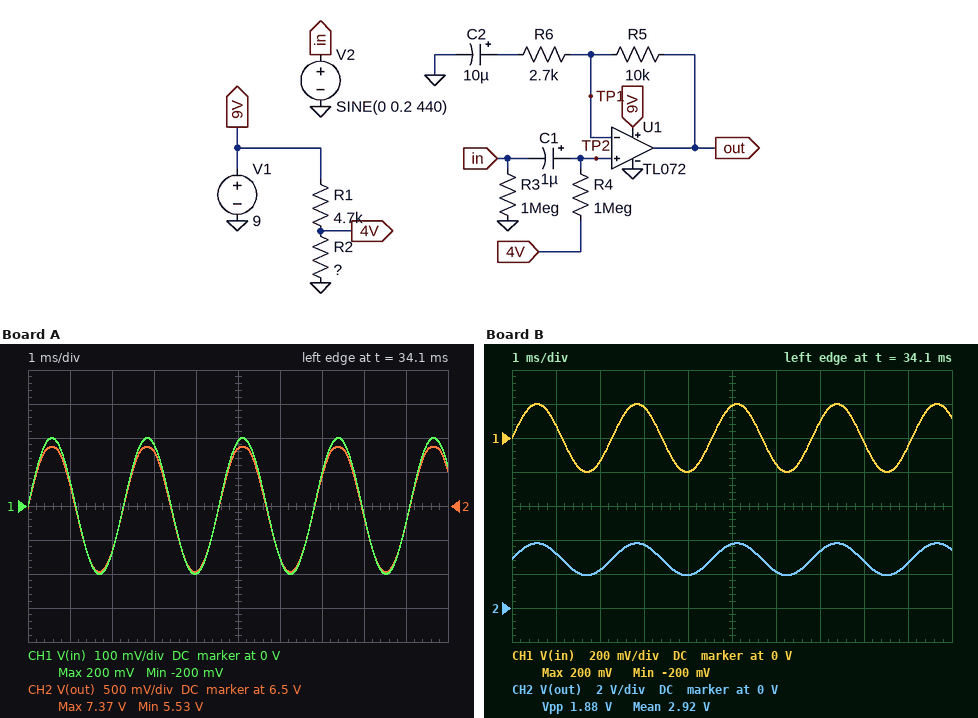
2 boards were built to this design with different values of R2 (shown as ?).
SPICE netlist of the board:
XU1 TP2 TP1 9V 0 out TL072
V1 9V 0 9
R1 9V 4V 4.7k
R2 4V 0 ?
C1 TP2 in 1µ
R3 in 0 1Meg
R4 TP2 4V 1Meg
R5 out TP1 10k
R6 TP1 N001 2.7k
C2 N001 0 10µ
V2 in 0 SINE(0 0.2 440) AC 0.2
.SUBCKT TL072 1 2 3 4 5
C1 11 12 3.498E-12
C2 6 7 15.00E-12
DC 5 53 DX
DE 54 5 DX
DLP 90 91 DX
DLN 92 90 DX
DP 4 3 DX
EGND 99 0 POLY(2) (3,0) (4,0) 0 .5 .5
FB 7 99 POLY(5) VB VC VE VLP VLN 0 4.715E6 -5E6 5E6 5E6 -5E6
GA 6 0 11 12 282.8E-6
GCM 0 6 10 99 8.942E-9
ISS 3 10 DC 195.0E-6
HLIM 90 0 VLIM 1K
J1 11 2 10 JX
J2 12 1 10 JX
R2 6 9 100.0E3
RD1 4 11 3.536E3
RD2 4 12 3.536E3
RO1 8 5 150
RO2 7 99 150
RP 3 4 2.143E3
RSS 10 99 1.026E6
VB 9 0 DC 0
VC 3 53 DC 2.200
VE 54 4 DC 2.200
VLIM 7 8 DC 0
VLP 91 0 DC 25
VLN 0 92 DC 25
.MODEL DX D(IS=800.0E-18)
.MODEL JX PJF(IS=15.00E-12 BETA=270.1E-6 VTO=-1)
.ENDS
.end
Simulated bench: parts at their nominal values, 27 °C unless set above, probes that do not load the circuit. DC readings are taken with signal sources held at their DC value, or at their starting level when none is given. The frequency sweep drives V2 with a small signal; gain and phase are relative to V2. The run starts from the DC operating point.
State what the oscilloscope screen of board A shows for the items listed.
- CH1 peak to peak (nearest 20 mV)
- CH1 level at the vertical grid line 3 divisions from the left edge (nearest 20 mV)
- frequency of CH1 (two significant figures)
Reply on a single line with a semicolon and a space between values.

400 mV; 180 mV; 440 Hz
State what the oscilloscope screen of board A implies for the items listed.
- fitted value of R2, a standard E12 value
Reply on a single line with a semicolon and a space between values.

12 kΩ
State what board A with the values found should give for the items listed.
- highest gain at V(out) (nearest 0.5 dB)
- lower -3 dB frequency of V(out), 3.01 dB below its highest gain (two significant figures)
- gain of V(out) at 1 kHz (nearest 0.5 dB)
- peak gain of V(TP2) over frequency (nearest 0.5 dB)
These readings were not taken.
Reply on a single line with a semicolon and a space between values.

13.5 dB; 5.6 Hz; 13.5 dB; 0 dB
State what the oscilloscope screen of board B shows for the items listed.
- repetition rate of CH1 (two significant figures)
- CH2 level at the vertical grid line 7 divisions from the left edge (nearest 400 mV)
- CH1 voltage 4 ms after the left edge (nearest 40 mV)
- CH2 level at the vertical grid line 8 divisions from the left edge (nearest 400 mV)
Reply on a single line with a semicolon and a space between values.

440 Hz; 3.2 V; -200 mV; 2.8 V
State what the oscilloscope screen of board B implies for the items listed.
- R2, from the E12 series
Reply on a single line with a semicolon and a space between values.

2.2 kΩ
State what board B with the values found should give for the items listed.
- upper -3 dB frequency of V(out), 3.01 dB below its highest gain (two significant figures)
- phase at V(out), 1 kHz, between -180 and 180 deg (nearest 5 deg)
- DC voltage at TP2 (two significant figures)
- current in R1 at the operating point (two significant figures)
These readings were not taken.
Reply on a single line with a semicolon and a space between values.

820 kHz; 0 deg; 2.9 V; 1.3 mA
